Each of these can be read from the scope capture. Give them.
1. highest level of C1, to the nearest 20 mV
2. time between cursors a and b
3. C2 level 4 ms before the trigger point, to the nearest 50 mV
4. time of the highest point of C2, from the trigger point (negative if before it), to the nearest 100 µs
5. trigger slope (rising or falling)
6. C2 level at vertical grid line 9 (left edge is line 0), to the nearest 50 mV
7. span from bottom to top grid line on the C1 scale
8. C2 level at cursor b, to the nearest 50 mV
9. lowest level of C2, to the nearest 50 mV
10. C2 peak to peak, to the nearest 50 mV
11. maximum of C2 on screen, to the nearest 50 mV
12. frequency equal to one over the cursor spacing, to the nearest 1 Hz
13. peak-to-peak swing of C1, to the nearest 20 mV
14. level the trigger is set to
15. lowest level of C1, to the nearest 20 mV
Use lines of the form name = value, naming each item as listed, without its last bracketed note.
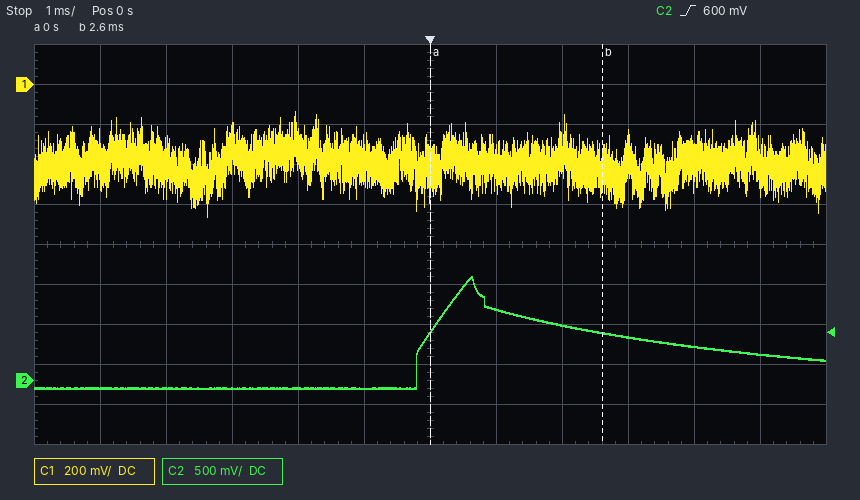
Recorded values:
highest level of C1, to the nearest 20 mV = -140 mV
time between cursors a and b = 2.6 ms
C2 level 4 ms before the trigger point, to the nearest 50 mV = -100 mV
time of the highest point of C2, from the trigger point (negative if before it), to the nearest 100 µs = +600 µs
trigger slope = rising
C2 level at vertical grid line 9 (left edge is line 0), to the nearest 50 mV = 550 mV
span from bottom to top grid line on the C1 scale = 2 V
C2 level at cursor b, to the nearest 50 mV = 600 mV
lowest level of C2, to the nearest 50 mV = -100 mV
C2 peak to peak, to the nearest 50 mV = 1.40 V
maximum of C2 on screen, to the nearest 50 mV = 1.30 V
frequency equal to one over the cursor spacing, to the nearest 1 Hz = 385 Hz
peak-to-peak swing of C1, to the nearest 20 mV = 520 mV
level the trigger is set to = 600 mV
lowest level of C1, to the nearest 20 mV = -660 mV
